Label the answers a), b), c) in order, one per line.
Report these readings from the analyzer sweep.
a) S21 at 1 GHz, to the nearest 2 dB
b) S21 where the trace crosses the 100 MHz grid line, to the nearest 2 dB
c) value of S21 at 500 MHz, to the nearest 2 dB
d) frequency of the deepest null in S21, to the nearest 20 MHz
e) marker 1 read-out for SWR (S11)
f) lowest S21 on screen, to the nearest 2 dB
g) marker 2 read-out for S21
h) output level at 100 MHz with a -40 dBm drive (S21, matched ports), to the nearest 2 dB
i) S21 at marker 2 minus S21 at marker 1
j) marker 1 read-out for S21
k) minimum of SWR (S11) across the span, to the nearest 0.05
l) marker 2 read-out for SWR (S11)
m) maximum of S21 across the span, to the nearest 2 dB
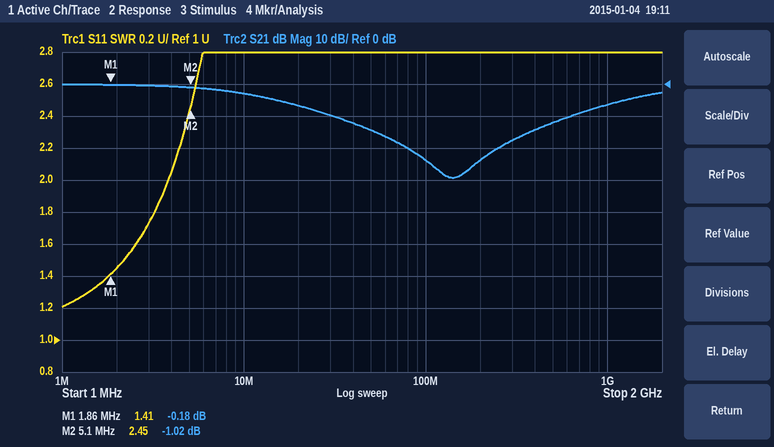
a) -6 dB
b) -24 dB
c) -12 dB
d) 140 MHz
e) 1.41
f) -30 dB
g) -1.02 dB
h) -64 dBm
i) -0.84 dB
j) -0.18 dB
k) 1.20
l) 2.45
m) 0 dB
